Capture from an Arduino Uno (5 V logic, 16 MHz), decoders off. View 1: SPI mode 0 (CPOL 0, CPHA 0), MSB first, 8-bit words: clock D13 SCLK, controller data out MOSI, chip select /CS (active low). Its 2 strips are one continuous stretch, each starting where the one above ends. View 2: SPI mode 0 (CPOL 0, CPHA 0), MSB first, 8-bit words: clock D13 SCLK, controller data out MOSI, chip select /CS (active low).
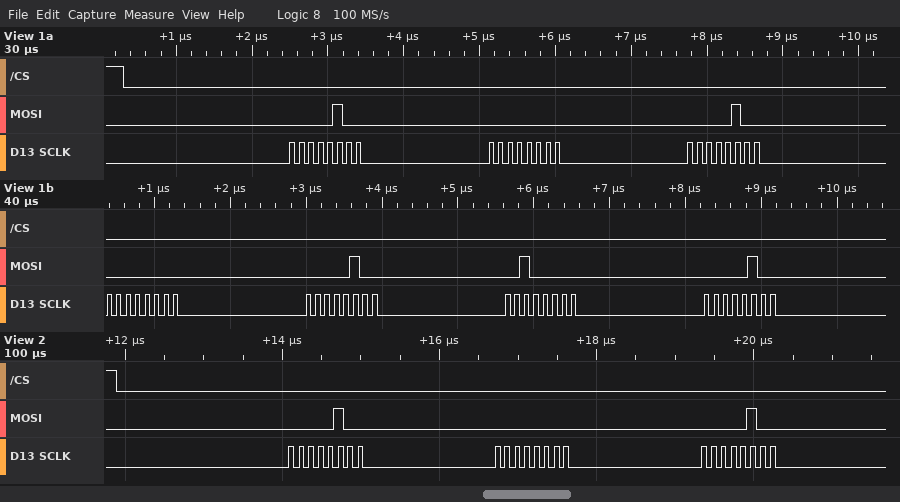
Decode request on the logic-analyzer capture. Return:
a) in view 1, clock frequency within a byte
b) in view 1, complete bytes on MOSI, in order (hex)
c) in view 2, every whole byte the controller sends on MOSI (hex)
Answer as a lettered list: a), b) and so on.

a) 8 MHz
b) 04 00 04 00 04 20 04
c) 04 00 04
